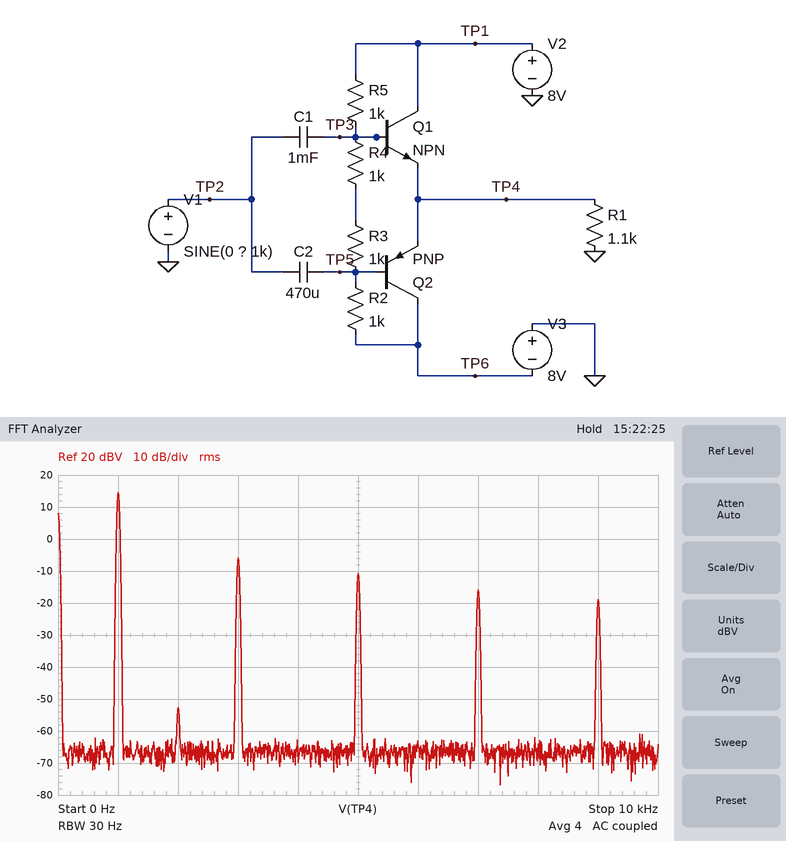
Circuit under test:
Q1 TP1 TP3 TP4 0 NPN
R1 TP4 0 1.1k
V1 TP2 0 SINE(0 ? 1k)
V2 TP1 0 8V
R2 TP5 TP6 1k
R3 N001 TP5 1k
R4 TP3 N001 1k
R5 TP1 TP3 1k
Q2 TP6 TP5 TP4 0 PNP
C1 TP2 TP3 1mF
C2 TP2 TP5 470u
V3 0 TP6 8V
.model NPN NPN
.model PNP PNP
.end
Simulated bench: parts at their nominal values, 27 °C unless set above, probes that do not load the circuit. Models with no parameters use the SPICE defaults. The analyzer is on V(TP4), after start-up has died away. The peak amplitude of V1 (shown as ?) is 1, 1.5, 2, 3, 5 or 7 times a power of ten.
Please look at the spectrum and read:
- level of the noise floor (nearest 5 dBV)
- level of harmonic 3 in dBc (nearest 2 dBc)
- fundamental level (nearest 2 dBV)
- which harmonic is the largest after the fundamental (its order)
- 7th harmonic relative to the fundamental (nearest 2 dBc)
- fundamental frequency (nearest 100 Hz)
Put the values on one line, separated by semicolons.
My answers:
-65 dBV; -20 dBc; 14 dBV; 3; -30 dBc; 1.0 kHz
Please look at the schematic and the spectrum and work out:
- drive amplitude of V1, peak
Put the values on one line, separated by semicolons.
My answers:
10 V
